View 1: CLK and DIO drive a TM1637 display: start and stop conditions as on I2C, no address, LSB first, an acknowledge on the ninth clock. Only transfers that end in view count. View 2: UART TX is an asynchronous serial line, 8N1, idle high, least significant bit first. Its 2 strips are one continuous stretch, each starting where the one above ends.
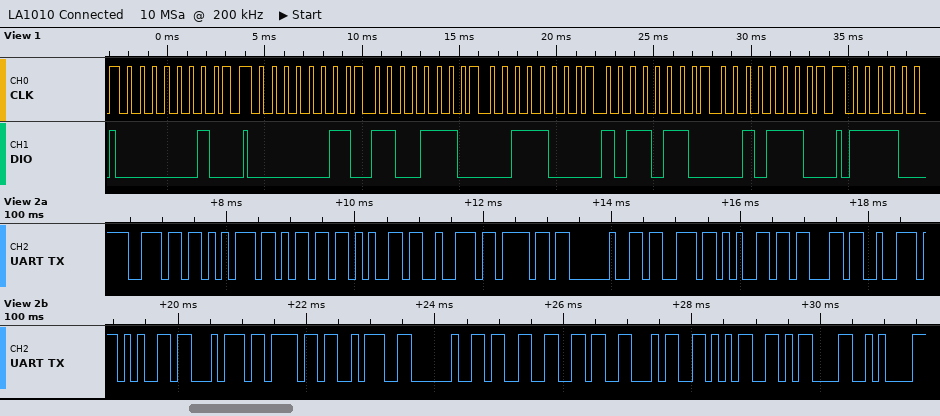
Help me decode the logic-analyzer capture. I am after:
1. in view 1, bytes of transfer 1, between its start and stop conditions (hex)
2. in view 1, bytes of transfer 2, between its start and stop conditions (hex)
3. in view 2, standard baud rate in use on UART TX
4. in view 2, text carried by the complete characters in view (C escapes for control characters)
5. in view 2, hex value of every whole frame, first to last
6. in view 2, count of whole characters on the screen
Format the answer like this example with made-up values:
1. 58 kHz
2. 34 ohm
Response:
1. 40
2. C0 73 1C 6D 74
3. 9600 baud
4. "numero secreto: 3645\r\n"
5. 6E 75 6D 65 72 6F 20 73 65 63 72 65 74 6F 3A 20 33 36 34 35 0D 0A
6. 22
